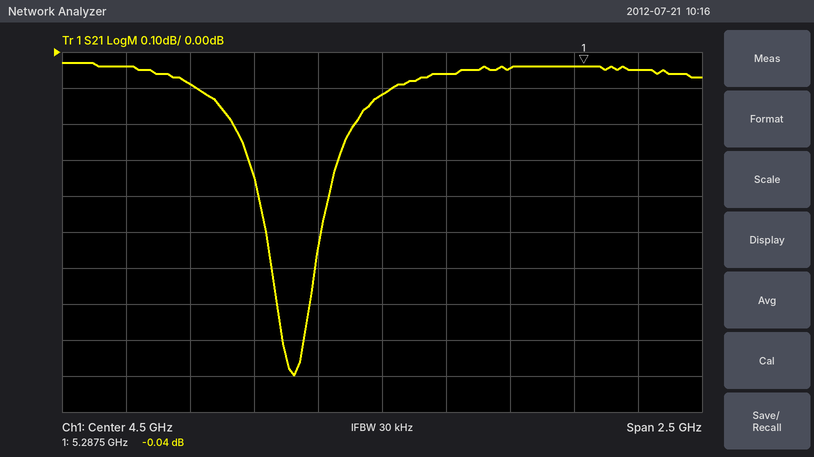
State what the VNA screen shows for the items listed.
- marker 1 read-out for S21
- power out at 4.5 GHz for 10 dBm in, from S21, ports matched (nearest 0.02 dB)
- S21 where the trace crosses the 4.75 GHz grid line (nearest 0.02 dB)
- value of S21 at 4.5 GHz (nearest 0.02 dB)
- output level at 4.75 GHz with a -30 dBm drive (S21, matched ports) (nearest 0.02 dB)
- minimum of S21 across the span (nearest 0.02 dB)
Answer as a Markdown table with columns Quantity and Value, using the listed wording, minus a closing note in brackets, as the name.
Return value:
| Quantity | Value |
|---|---|
| marker 1 read-out for S21 | -0.04 dB |
| power out at 4.5 GHz for 10 dBm in, from S21, ports matched | 9.88 dBm |
| S21 where the trace crosses the 4.75 GHz grid line | -0.06 dB |
| value of S21 at 4.5 GHz | -0.12 dB |
| output level at 4.75 GHz with a -30 dBm drive (S21, matched ports) | -30.06 dBm |
| minimum of S21 across the span | -0.90 dB |
